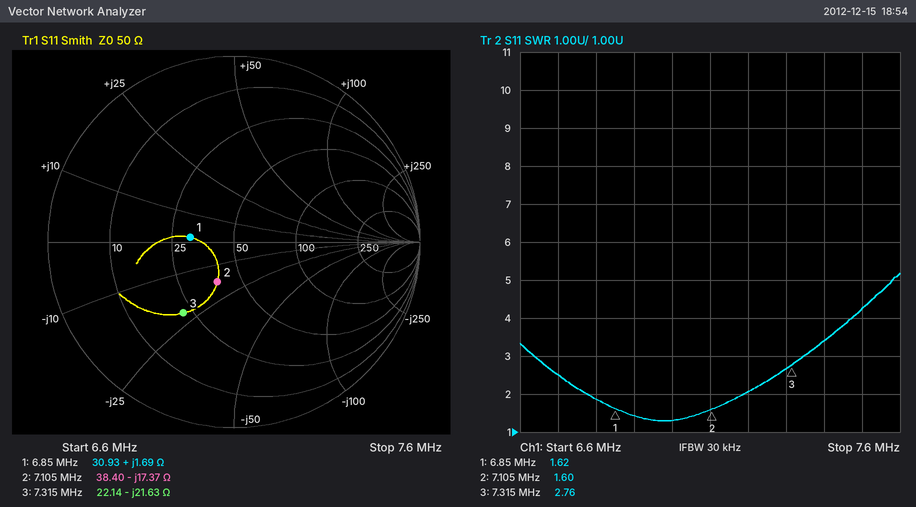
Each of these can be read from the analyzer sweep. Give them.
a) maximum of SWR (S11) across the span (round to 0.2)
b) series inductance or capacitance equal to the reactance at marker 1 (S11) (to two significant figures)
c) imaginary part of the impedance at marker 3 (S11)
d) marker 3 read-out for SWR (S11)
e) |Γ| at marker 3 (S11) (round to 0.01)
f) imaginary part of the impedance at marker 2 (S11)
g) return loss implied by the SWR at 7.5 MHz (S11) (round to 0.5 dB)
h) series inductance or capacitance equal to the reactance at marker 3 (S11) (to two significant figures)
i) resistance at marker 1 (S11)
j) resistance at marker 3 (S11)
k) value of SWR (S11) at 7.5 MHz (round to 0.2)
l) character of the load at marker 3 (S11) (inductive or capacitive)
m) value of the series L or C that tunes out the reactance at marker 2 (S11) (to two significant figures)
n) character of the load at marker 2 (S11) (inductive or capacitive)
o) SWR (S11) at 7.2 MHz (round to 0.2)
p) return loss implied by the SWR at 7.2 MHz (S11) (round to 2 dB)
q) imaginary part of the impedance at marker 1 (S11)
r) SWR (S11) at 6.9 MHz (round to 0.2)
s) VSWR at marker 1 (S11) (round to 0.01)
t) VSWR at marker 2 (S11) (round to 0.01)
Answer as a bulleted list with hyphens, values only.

- 5.2
- 39 nH
- -21.63 Ω
- 2.76
- 0.47
- -17.37 Ω
- 4.0 dB
- 1.0 nF
- 30.93 Ω
- 22.14 Ω
- 4.2
- capacitive
- 390 nH
- capacitive
- 2.0
- 10 dB
- +1.69 Ω
- 1.4
- 1.62
- 1.60
